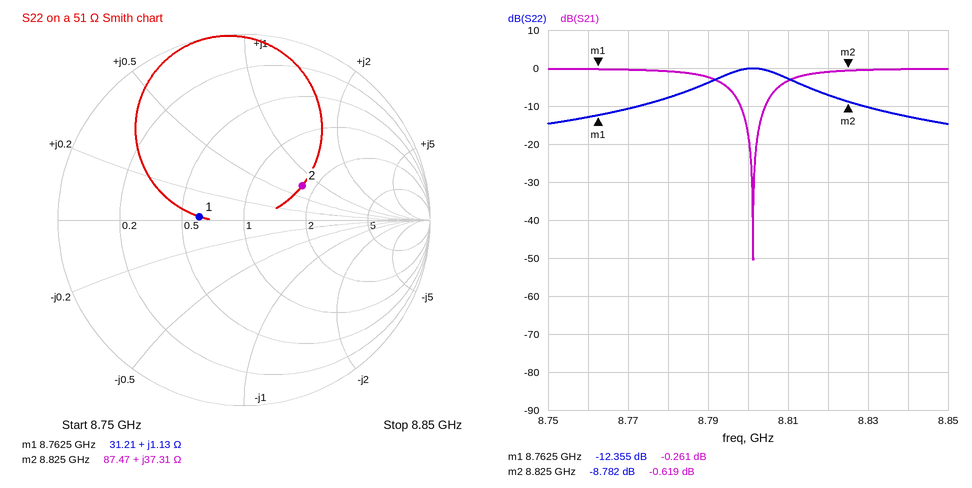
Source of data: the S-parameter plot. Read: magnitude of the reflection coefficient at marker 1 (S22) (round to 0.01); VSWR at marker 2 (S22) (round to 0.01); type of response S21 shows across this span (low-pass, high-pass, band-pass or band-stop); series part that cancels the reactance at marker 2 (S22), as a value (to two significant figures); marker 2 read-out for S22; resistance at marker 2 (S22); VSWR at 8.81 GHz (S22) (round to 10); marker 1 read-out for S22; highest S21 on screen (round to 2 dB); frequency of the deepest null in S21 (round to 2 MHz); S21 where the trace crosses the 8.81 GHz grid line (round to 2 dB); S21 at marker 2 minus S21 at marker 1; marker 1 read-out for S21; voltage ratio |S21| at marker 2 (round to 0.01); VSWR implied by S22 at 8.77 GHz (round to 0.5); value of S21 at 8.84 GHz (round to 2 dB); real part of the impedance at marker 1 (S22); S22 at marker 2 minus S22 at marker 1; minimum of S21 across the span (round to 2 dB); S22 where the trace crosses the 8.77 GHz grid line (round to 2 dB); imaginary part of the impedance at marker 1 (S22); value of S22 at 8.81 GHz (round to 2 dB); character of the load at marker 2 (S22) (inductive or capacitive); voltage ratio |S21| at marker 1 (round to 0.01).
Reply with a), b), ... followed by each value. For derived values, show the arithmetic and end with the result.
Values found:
a) 0.24
b) (1 + 0.3638)/(1 − 0.3638) ≈ 2.14
c) band-stop
d) C = 1/(2π × 8.825 GHz × 37.31 Ω) ≈ 483 fF, so 480 fF to two significant figures
e) -8.782 dB
f) 87.47 Ω
g) |Γ| = 10^(-2/20) = 0.7943; VSWR = (1 + 0.7943)/(1 − 0.7943) ≈ 8.72, so 10 to the nearest 10
h) -12.355 dB
i) 0 dB
j) 8.802 GHz
k) -4 dB
l) -0.619 − (-0.261) = -0.358 dB
m) -0.261 dB
n) 10^(-0.619/20) ≈ 0.93
o) |Γ| = 10^(-10/20) = 0.3162; VSWR = (1 + 0.3162)/(1 − 0.3162) ≈ 1.92, so 2.0 to the nearest 0.5
p) 0 dB
q) 31.21 Ω
r) -8.782 − (-12.355) = 3.573 dB
s) -50 dB
t) -10 dB
u) +1.13 Ω
v) -2 dB
w) inductive
x) 10^(-0.261/20) ≈ 0.97
